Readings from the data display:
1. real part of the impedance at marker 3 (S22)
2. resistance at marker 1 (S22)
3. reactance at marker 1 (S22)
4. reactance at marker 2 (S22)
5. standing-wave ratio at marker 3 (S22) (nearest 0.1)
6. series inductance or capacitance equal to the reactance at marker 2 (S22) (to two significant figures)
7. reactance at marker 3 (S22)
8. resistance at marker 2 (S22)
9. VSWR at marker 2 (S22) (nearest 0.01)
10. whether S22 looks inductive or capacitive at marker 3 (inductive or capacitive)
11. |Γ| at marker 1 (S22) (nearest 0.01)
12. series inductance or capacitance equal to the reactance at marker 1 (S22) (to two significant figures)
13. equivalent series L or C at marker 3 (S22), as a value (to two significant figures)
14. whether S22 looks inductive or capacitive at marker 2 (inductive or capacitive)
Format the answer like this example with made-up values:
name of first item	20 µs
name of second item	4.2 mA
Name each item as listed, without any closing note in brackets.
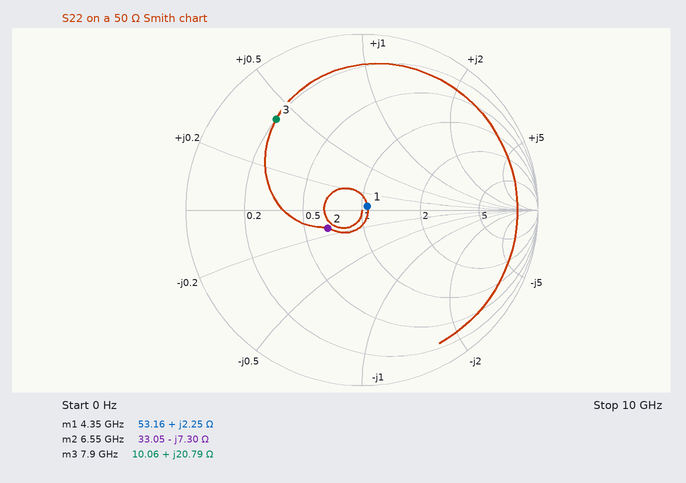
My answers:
real part of the impedance at marker 3	10.06 Ω
resistance at marker 1	53.16 Ω
reactance at marker 1	+2.25 Ω
reactance at marker 2	-7.30 Ω
standing-wave ratio at marker 3 (S22)	5.9
series inductance or capacitance equal to the reactance at marker 2 (S22)	3.3 pF
reactance at marker 3	+20.79 Ω
resistance at marker 2	33.05 Ω
VSWR at marker 2 (S22)	1.57
whether S22 looks inductive or capacitive at marker 3	inductive
|Γ| at marker 1 (S22)	0.04
series inductance or capacitance equal to the reactance at marker 1 (S22)	82 pH
equivalent series L or C at marker 3 (S22), as a value	420 pH
whether S22 looks inductive or capacitive at marker 2	capacitive
